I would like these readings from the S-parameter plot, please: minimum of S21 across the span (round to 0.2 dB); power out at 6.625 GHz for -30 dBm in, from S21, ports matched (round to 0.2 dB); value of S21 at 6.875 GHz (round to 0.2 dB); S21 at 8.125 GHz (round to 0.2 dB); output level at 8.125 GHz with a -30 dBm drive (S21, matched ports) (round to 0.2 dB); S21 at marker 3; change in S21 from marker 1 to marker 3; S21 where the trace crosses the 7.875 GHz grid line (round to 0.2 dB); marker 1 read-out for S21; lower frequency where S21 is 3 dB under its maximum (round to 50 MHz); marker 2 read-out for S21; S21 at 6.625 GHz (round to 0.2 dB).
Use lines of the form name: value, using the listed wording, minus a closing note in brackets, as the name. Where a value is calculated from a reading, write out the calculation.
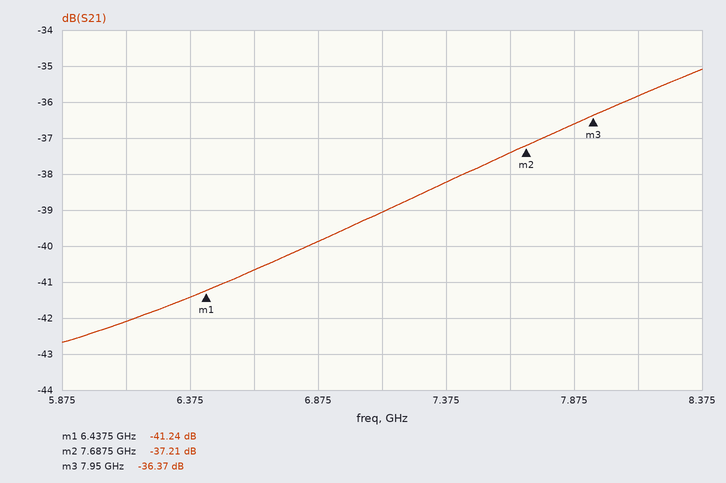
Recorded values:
minimum of S21 across the span: -42.6 dB
power out at 6.625 GHz for -30 dBm in, from S21, ports matched: -30 dBm + (-40.6 dB) = -70.6 dBm
value of S21 at 6.875 GHz: -39.8 dB
S21 at 8.125 GHz: -35.8 dB
output level at 8.125 GHz with a -30 dBm drive (S21, matched ports): -30 dBm + (-35.8 dB) = -65.8 dBm
S21 at marker 3: -36.37 dB
change in S21 from marker 1 to marker 3: -36.37 − (-41.24) = 4.87 dB
S21 where the trace crosses the 7.875 GHz grid line: -36.6 dB
marker 1 read-out for S21: -41.24 dB
lower frequency where S21 is 3 dB under its maximum: 7.40 GHz
marker 2 read-out for S21: -37.21 dB
S21 at 6.625 GHz: -40.6 dB
